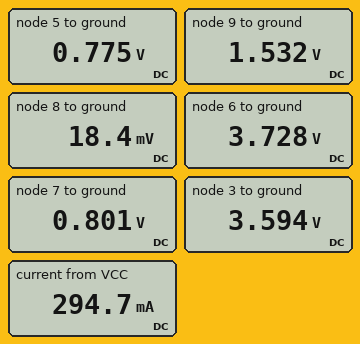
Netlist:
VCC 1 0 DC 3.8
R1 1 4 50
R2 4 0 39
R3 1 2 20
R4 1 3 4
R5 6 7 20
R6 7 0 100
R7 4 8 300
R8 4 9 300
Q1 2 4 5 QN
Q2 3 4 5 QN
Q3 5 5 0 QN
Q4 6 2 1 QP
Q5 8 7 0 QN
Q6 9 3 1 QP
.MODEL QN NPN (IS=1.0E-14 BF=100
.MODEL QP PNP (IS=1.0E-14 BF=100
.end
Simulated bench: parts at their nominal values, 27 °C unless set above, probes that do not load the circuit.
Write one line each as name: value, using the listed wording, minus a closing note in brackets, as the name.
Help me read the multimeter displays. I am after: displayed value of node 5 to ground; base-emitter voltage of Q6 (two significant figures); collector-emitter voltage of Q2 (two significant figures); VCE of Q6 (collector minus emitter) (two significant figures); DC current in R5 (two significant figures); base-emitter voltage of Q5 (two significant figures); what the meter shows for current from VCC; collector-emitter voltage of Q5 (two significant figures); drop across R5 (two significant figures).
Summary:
displayed value of node 5 to ground: 0.775 V
base-emitter voltage of Q6: -210 mV
collector-emitter voltage of Q2: 2.8 V
VCE of Q6 (collector minus emitter): -2.3 V
DC current in R5: 150 mA
base-emitter voltage of Q5: 800 mV
what the meter shows for current from VCC: 294.7 mA
collector-emitter voltage of Q5: 18 mV
drop across R5: 2.9 V
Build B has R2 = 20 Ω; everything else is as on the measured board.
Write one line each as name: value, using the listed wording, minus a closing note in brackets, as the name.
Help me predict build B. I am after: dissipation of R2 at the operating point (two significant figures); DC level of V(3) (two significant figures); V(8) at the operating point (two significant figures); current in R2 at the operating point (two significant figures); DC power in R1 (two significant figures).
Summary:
dissipation of R2 at the operating point: 59 mW
DC level of V(3): 3.8 V
V(8) at the operating point: 1.1 V
current in R2 at the operating point: 54 mA
DC power in R1: 150 mW
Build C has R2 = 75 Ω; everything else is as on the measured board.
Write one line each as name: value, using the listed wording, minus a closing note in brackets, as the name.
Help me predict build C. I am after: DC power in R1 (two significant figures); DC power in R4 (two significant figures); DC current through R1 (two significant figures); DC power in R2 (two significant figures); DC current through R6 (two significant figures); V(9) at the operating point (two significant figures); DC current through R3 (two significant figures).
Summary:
DC power in R1: 89 mW
DC power in R4: 180 mW
DC current through R1: 42 mA
DC power in R2: 38 mW
DC current through R6: 8.0 mA
V(9) at the operating point: 3.8 V
DC current through R3: 43 mA
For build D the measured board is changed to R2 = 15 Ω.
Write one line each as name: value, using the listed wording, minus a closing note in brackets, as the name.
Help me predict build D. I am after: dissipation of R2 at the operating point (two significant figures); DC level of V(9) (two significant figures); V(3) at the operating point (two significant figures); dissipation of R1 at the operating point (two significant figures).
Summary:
dissipation of R2 at the operating point: 51 mW
DC level of V(9): 880 mV
V(3) at the operating point: 3.8 V
dissipation of R1 at the operating point: 170 mW
